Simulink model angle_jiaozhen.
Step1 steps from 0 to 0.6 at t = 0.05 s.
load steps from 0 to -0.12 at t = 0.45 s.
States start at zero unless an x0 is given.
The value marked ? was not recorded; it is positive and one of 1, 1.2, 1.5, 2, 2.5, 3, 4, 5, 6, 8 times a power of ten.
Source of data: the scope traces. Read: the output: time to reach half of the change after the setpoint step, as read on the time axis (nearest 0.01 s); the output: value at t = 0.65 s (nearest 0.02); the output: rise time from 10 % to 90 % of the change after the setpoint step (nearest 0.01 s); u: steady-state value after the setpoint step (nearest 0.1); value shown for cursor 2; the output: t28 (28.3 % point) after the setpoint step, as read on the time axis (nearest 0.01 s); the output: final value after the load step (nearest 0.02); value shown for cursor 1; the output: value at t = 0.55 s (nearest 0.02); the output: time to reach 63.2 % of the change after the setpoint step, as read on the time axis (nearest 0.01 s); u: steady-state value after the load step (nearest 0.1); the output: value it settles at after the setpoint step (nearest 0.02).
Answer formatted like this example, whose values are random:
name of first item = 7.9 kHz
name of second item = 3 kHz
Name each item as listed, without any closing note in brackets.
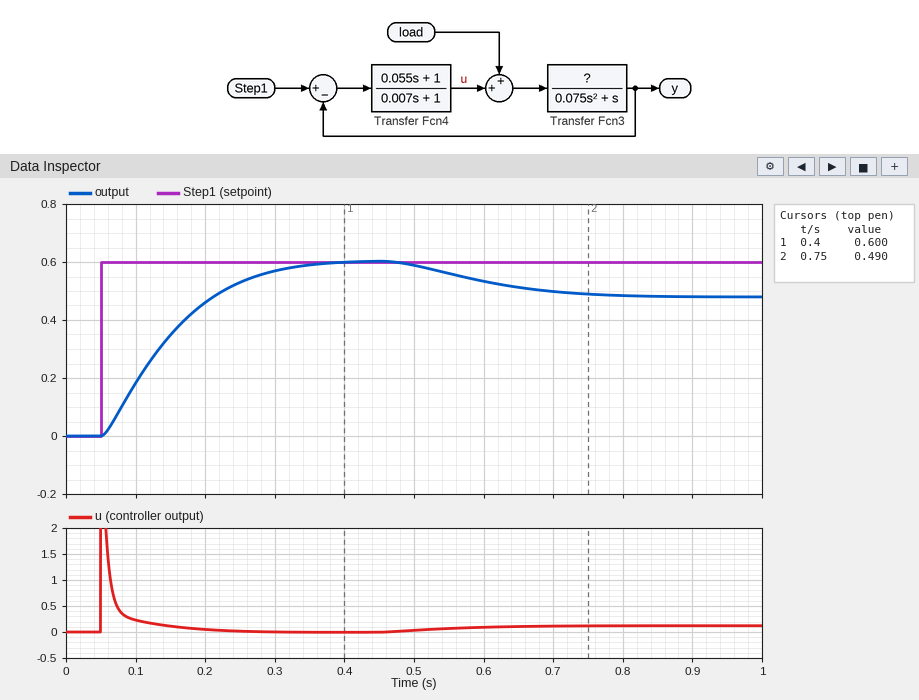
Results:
the output: time to reach half of the change after the setpoint step, as read on the time axis = 0.13 s
the output: value at t = 0.65 s = 0.52
the output: rise time from 10 % to 90 % of the change after the setpoint step = 0.19 s
u: steady-state value after the setpoint step = 0.0
value shown for cursor 2 = 0.490
the output: t28 (28.3 % point) after the setpoint step, as read on the time axis = 0.10 s
the output: final value after the load step = 0.48
value shown for cursor 1 = 0.600
the output: value at t = 0.55 s = 0.56
the output: time to reach 63.2 % of the change after the setpoint step, as read on the time axis = 0.16 s
u: steady-state value after the load step = 0.1
the output: value it settles at after the setpoint step = 0.60
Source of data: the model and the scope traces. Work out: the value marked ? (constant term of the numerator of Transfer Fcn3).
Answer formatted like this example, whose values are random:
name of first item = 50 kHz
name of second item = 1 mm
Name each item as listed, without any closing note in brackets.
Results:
the value marked ? = 10
